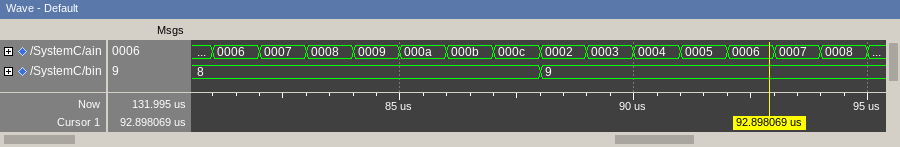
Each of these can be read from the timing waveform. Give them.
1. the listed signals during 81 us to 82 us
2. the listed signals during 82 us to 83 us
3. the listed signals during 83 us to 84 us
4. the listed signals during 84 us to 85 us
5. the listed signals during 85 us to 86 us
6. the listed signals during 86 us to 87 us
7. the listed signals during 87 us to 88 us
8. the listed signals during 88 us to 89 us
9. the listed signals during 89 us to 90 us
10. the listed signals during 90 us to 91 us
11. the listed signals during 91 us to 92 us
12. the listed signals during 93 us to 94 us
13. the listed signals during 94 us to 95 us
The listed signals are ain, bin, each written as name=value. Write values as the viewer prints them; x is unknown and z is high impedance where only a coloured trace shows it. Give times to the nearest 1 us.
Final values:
ain=0006, bin=8
ain=0007, bin=8
ain=0008, bin=8
ain=0009, bin=8
ain=000a, bin=8
ain=000b, bin=8
ain=000c, bin=8
ain=0002, bin=9
ain=0003, bin=9
ain=0004, bin=9
ain=0005, bin=9
ain=0007, bin=9
ain=0008, bin=9
